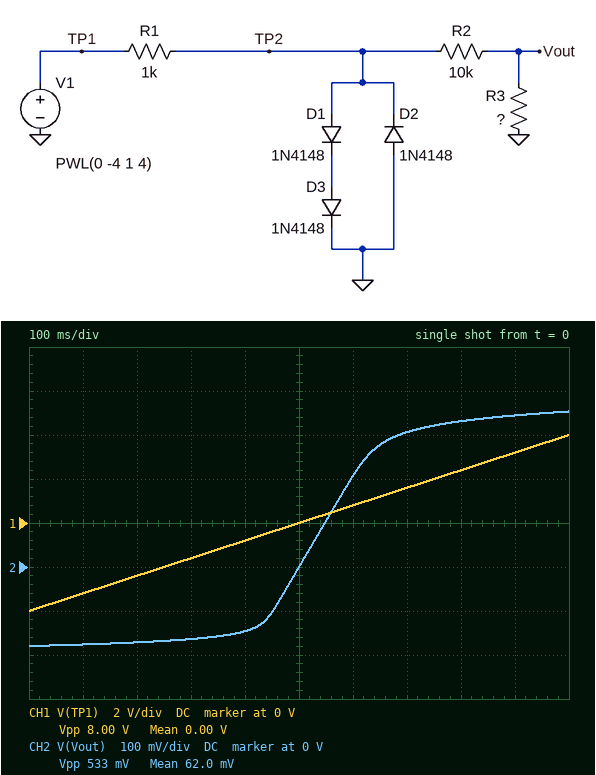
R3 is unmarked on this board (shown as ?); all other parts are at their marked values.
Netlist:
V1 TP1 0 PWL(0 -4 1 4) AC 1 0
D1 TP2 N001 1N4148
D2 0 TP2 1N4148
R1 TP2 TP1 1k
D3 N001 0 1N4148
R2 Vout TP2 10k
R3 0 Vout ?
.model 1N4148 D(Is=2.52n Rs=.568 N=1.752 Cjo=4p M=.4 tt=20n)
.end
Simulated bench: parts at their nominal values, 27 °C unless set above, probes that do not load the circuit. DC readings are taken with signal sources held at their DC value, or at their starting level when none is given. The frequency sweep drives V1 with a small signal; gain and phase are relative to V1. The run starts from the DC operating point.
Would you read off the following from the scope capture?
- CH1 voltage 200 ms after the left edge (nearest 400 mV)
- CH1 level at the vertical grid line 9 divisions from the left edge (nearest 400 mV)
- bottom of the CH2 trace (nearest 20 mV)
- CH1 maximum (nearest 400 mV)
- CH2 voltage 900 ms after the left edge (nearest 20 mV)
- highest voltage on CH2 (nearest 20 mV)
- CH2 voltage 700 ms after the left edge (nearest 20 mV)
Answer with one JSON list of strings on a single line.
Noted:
["-2.4 V", "3.2 V", "-180 mV", "4.0 V", "340 mV", "360 mV", "300 mV"]
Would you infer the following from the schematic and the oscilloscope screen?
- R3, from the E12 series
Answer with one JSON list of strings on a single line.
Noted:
["3.9 kΩ"]
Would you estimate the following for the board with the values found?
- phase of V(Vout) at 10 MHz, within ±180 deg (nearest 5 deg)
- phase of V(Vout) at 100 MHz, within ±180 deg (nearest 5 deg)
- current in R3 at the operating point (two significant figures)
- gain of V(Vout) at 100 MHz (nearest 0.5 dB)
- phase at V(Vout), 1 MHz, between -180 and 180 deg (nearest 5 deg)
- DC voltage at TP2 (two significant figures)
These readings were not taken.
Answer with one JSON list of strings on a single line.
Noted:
["-50 deg", "-60 deg", "46 µA", "-69.0 dB", "-5 deg", "-640 mV"]
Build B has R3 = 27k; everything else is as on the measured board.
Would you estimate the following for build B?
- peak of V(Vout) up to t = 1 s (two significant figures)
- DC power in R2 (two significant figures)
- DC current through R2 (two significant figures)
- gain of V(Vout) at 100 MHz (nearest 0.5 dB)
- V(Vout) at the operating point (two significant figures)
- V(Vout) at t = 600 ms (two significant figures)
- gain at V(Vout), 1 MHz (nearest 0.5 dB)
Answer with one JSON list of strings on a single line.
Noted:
["920 mV", "3.0 µW", "17 µA", "-61.0 dB", "-470 mV", "560 mV", "-40.0 dB"]
